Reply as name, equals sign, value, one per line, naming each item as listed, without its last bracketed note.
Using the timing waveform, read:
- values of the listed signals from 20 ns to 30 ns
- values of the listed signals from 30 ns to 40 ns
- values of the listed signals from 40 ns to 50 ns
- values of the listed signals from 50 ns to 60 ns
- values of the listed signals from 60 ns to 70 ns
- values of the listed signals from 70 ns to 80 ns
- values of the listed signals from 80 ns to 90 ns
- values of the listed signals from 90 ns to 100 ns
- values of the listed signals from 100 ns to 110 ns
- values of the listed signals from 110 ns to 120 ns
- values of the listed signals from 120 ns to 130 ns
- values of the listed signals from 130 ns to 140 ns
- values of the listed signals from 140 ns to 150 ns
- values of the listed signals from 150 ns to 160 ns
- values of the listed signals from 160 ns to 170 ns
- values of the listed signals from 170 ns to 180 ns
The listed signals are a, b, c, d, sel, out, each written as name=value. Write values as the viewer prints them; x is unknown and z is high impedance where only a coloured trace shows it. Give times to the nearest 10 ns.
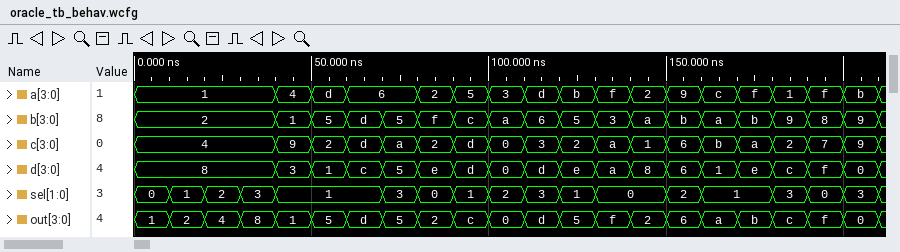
values of the listed signals from 20 ns to 30 ns = a=1, b=2, c=4, d=8, sel=2, out=4
values of the listed signals from 30 ns to 40 ns = a=1, b=2, c=4, d=8, sel=3, out=8
values of the listed signals from 40 ns to 50 ns = a=4, b=1, c=9, d=3, sel=1, out=1
values of the listed signals from 50 ns to 60 ns = a=d, b=5, c=2, d=1, sel=1, out=5
values of the listed signals from 60 ns to 70 ns = a=6, b=d, c=d, d=c, sel=1, out=d
values of the listed signals from 70 ns to 80 ns = a=6, b=5, c=a, d=5, sel=3, out=5
values of the listed signals from 80 ns to 90 ns = a=2, b=f, c=2, d=e, sel=0, out=2
values of the listed signals from 90 ns to 100 ns = a=5, b=c, c=d, d=d, sel=1, out=c
values of the listed signals from 100 ns to 110 ns = a=3, b=a, c=0, d=0, sel=2, out=0
values of the listed signals from 110 ns to 120 ns = a=d, b=6, c=3, d=d, sel=3, out=d
values of the listed signals from 120 ns to 130 ns = a=b, b=5, c=2, d=e, sel=1, out=5
values of the listed signals from 130 ns to 140 ns = a=f, b=3, c=a, d=a, sel=0, out=f
values of the listed signals from 140 ns to 150 ns = a=2, b=a, c=1, d=8, sel=0, out=2
values of the listed signals from 150 ns to 160 ns = a=9, b=b, c=6, d=6, sel=2, out=6
values of the listed signals from 160 ns to 170 ns = a=c, b=a, c=b, d=1, sel=1, out=a
values of the listed signals from 170 ns to 180 ns = a=f, b=b, c=a, d=e, sel=1, out=b
